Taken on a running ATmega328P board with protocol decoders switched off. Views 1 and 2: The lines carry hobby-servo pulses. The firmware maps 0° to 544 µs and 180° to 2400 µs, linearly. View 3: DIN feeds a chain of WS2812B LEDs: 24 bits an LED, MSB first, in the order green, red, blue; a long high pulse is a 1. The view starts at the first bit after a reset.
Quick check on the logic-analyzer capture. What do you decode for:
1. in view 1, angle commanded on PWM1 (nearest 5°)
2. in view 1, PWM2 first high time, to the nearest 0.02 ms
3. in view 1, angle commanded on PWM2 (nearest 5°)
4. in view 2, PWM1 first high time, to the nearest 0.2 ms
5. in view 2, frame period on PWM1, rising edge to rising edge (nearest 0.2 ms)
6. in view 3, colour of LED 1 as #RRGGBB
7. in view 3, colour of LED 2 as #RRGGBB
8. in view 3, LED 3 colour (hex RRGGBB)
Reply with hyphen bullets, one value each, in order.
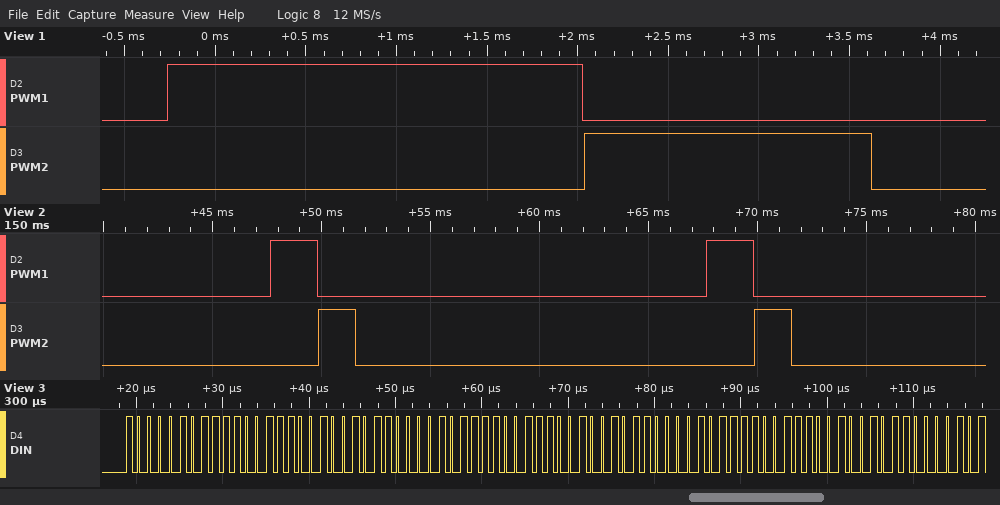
- 170°
- 1.58 ms
- 100°
- 2.2 ms
- 20.0 ms
- #E78525
- #E78525
- #E78525
